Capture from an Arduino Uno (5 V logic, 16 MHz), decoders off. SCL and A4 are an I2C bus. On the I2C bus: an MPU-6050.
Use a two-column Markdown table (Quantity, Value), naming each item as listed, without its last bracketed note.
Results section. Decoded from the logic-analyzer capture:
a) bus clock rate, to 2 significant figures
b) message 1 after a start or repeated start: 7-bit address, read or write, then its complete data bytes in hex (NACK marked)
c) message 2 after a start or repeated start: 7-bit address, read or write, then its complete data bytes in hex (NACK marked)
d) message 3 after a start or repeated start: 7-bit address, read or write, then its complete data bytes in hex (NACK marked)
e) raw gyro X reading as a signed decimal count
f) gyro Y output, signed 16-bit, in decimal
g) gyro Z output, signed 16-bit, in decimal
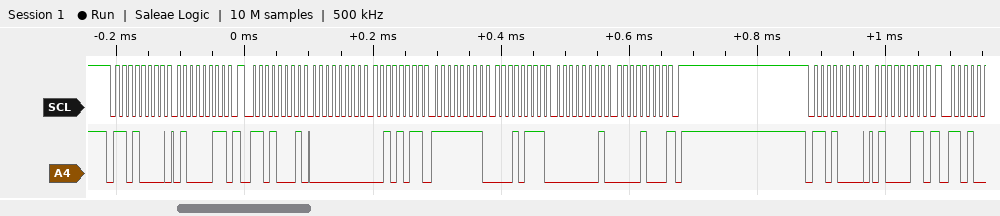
| Quantity | Value |
|---|---|
| bus clock rate, to 2 significant figures | 100 kHz |
| message 1 after a start or repeated start: 7-bit address, read or write, then its complete data bytes in hex | 0x68 write: 43 |
| message 2 after a start or repeated start: 7-bit address, read or write, then its complete data bytes in hex | 0x68 read: 00 2B FF 17 01 08 NACK |
| message 3 after a start or repeated start: 7-bit address, read or write, then its complete data bytes in hex | 0x68 write: 43 |
| raw gyro X reading as a signed decimal count | 43 |
| gyro Y output, signed 16-bit, in decimal | -233 |
| gyro Z output, signed 16-bit, in decimal | 264 |
